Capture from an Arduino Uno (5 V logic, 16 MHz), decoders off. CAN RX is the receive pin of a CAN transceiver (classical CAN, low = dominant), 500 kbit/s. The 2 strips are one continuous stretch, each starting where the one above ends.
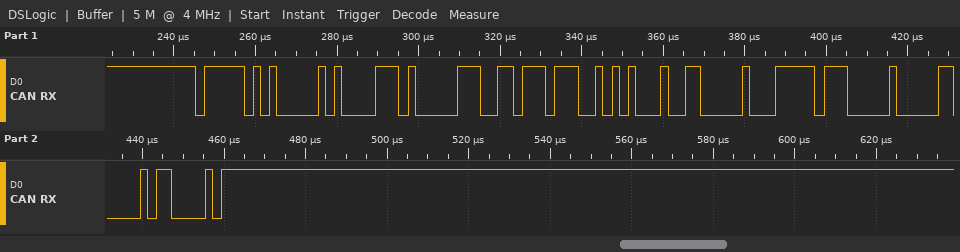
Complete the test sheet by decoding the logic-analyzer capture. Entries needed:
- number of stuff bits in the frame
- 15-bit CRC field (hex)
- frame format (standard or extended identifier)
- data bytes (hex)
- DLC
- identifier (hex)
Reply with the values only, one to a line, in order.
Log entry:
7
0x10B0
standard
74 19 BB 95 13 00 FF 00
8
0x7E8
